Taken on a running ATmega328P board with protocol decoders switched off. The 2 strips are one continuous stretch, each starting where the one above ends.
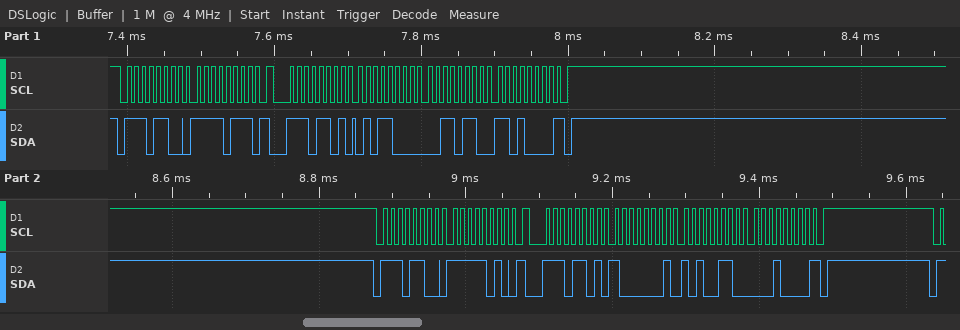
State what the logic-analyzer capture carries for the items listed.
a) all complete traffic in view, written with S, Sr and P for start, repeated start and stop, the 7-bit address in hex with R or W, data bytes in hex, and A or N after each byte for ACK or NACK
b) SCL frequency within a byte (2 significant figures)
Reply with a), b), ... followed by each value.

a) S 76W A F7 A Sr 76R A 58 A 36 A D0 N P S 76W A FA A Sr 76R A 81 A A6 A 10 N P
b) 100 kHz
